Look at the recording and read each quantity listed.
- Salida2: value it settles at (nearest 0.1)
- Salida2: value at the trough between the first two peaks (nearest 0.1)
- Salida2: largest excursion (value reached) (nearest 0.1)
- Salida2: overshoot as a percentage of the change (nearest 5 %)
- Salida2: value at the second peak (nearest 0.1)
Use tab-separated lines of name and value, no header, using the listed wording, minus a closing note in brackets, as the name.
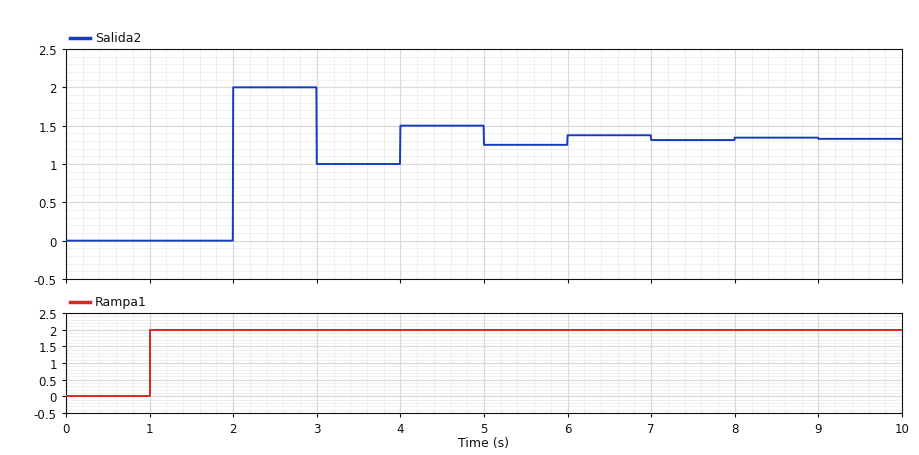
Salida2: value it settles at	1.3
Salida2: value at the trough between the first two peaks	1.0
Salida2: largest excursion (value reached)	2.0
Salida2: overshoot as a percentage of the change	50 %
Salida2: value at the second peak	1.5
